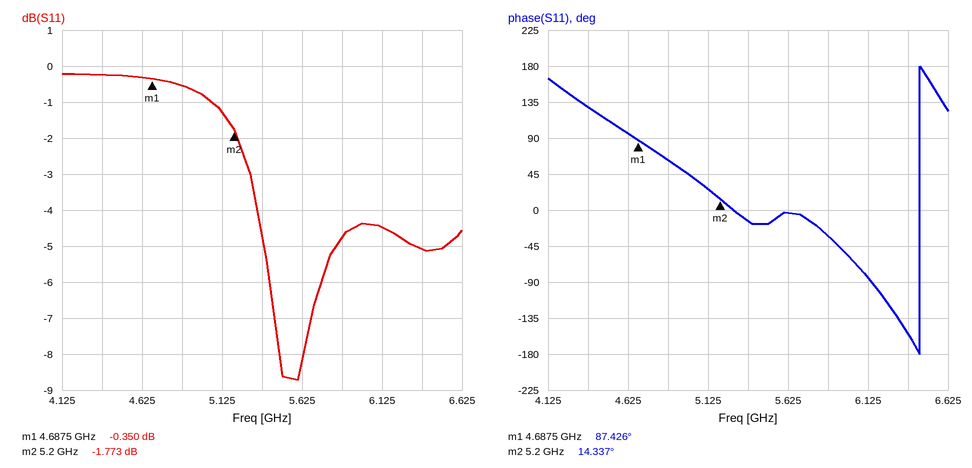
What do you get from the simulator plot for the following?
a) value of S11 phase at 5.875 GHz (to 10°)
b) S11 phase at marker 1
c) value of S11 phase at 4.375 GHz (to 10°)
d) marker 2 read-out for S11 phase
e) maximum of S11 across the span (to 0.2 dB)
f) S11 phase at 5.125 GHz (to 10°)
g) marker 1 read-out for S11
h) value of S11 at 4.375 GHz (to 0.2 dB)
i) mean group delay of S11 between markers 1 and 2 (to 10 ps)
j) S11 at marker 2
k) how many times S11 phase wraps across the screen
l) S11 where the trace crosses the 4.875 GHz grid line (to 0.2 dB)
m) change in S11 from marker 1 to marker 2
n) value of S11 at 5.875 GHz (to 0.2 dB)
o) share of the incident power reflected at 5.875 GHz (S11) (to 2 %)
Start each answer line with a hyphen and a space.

- -30°
- 87.426°
- 130°
- 14.337°
- -0.2 dB
- 30°
- -0.350 dB
- -0.2 dB
- 400 ps
- -1.773 dB
- 1
- -0.6 dB
- -1.423 dB
- -4.8 dB
- 34 %
